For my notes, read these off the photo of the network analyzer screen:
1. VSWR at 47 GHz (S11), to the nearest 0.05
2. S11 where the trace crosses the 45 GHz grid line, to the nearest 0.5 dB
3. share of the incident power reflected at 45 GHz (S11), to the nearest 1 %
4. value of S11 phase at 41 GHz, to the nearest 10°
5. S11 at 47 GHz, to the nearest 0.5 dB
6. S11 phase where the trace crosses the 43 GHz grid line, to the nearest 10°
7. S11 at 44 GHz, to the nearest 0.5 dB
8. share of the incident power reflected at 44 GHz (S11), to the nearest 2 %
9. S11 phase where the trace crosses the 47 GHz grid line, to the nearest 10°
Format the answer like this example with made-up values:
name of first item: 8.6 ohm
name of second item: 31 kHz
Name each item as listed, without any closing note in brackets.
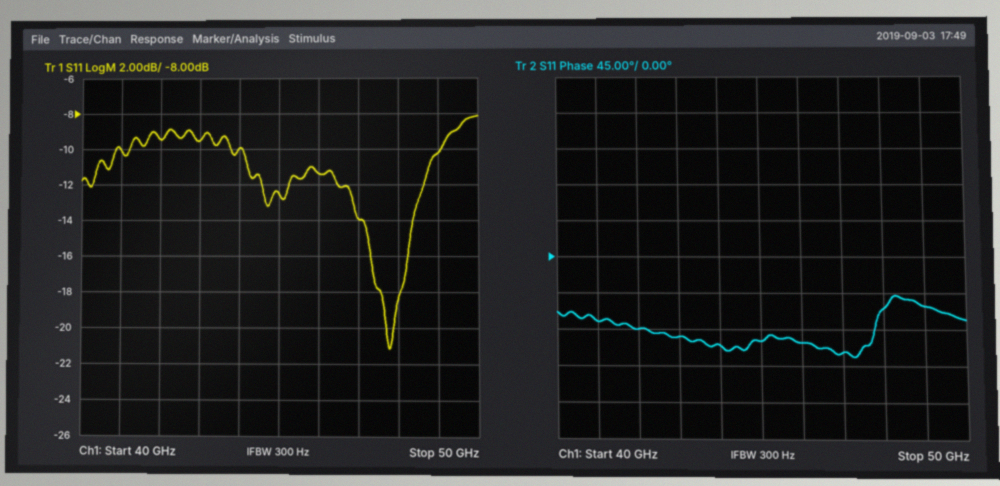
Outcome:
VSWR at 47 GHz (S11), to the nearest 0.05: 1.50
S11 where the trace crosses the 45 GHz grid line, to the nearest 0.5 dB: -12.5 dB
share of the incident power reflected at 45 GHz (S11), to the nearest 1 %: 6 %
value of S11 phase at 41 GHz, to the nearest 10°: -80°
S11 at 47 GHz, to the nearest 0.5 dB: -14.0 dB
S11 phase where the trace crosses the 43 GHz grid line, to the nearest 10°: -100°
S11 at 44 GHz, to the nearest 0.5 dB: -10.0 dB
share of the incident power reflected at 44 GHz (S11), to the nearest 2 %: 10 %
S11 phase where the trace crosses the 47 GHz grid line, to the nearest 10°: -120°
